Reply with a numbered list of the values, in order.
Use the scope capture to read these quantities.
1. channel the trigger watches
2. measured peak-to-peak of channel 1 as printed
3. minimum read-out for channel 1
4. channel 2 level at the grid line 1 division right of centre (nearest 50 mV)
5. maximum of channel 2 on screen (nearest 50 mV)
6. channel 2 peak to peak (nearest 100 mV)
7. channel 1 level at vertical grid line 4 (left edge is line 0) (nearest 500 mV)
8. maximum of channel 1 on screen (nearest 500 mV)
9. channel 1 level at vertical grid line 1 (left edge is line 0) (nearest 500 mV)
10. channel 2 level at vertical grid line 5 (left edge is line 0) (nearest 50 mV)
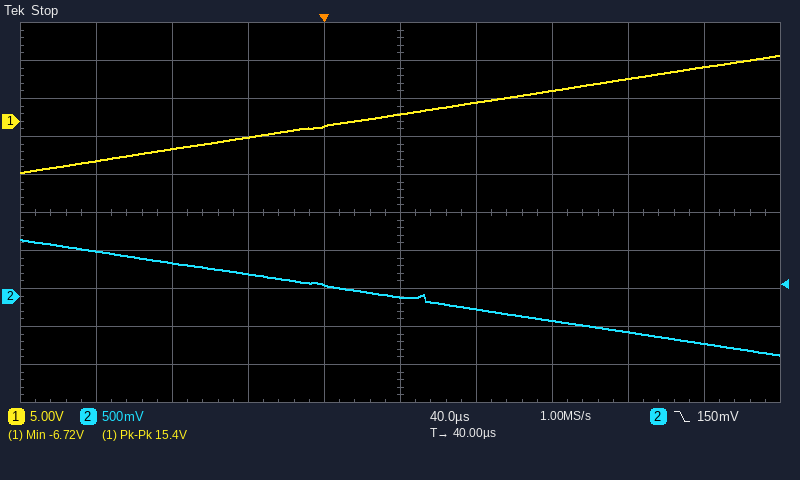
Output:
1. channel 2
2. 15.4 V
3. -6.72 V
4. -150 mV
5. 750 mV
6. 1.50 V
7. -500 mV
8. 8.5 V
9. -5.0 V
10. 0 mV
